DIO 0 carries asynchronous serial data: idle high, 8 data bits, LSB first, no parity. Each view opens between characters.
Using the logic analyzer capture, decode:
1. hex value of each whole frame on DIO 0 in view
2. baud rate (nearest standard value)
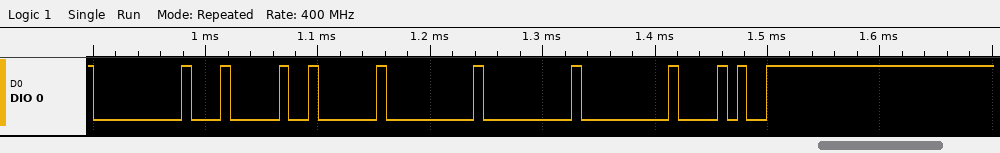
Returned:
00, 04, 02, 00, 00, 00, 28
115200 baud
